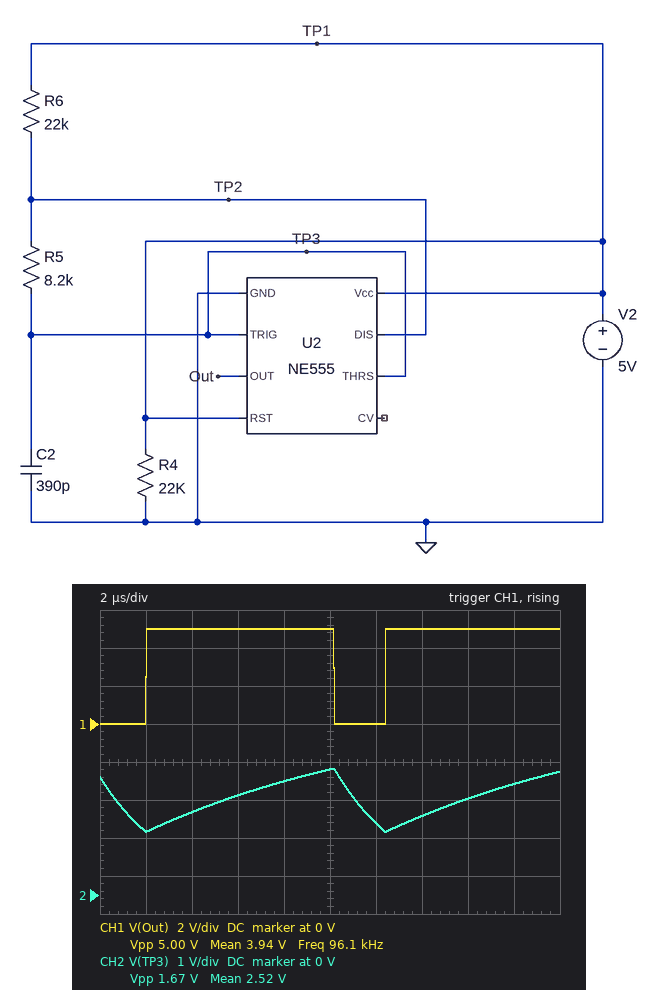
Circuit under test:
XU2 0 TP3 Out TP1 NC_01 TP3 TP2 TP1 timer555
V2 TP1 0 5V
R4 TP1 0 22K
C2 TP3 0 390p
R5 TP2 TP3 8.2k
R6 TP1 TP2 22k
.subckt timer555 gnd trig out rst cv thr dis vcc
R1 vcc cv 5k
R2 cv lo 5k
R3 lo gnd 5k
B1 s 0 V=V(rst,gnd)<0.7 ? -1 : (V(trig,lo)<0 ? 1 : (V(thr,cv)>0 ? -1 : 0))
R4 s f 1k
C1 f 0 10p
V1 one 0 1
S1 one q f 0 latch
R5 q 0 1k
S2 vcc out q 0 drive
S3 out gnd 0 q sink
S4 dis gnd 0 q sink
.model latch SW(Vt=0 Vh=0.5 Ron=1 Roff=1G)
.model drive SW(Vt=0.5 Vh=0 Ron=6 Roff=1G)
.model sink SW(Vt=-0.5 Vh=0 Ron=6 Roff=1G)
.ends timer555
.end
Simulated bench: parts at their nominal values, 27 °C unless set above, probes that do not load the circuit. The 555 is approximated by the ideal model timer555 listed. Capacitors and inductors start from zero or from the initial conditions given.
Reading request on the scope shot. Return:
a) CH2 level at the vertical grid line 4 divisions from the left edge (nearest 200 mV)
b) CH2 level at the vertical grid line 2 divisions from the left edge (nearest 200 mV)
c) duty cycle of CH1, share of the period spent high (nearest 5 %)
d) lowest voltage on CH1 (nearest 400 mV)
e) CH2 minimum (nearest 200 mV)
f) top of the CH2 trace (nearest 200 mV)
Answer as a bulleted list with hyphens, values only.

- 3.0 V
- 2.2 V
- 80 %
- 0 V
- 1.6 V
- 3.4 V
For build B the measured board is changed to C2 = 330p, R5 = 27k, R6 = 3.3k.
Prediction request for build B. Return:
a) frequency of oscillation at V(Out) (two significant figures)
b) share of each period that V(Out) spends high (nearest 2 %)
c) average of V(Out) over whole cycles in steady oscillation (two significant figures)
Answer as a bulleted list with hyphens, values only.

- 76 kHz
- 52 %
- 2.6 V
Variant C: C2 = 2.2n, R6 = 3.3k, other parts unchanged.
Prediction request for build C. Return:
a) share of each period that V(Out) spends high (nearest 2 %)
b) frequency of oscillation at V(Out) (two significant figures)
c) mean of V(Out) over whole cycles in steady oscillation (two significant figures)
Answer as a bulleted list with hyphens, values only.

- 58 %
- 33 kHz
- 2.9 V
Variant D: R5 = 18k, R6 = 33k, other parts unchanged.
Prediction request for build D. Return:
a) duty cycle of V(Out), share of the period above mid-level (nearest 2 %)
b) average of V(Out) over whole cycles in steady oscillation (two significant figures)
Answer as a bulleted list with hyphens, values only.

- 74 %
- 3.7 V
